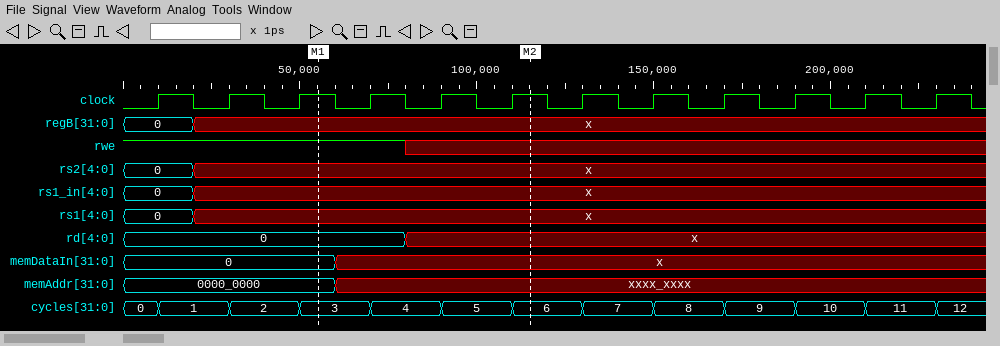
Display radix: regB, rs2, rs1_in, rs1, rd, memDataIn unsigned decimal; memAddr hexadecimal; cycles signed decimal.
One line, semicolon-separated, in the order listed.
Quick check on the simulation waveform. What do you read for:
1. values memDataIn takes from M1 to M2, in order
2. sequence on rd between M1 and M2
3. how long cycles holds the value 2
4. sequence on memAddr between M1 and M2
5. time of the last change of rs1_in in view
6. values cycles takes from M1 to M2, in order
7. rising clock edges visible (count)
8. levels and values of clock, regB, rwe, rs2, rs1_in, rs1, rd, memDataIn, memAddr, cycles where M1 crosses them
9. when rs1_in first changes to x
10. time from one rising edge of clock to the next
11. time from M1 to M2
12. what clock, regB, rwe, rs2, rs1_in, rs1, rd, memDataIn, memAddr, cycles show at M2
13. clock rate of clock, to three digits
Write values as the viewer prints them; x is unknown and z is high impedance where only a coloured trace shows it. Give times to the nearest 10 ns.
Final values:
0, x; 0, x; 20 ns; 0000_0000, xxxx_xxxx; 20 ns; 3, 4, 5, 6; 12; clock=1, regB=x, rwe=1, rs2=x, rs1_in=x, rs1=x, rd=0, memDataIn=0, memAddr=0000_0000, cycles=3; 20 ns; 20 ns; 60 ns; clock=1, regB=x, rwe=x, rs2=x, rs1_in=x, rs1=x, rd=x, memDataIn=x, memAddr=xxxx_xxxx, cycles=6; 50.0 MHz
